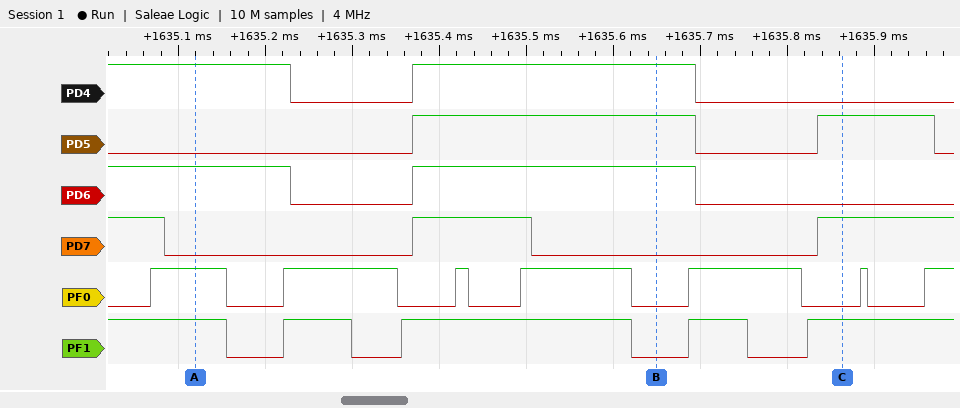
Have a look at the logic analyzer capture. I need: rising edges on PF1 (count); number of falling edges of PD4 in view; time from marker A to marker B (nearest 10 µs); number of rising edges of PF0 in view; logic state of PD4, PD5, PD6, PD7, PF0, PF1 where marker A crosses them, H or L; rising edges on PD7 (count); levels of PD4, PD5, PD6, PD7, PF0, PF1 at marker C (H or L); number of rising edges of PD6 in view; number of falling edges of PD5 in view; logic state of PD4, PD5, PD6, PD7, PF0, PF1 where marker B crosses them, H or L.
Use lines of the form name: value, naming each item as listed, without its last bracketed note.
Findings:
rising edges on PF1: 4
number of falling edges of PD4 in view: 2
time from marker A to marker B: 530 µs
number of rising edges of PF0 in view: 7
logic state of PD4, PD5, PD6, PD7, PF0, PF1 where marker A crosses them, H or L: PD4=H, PD5=L, PD6=H, PD7=L, PF0=H, PF1=H
rising edges on PD7: 2
levels of PD4, PD5, PD6, PD7, PF0, PF1 at marker C: PD4=L, PD5=H, PD6=L, PD7=H, PF0=L, PF1=H
number of rising edges of PD6 in view: 1
number of falling edges of PD5 in view: 2
logic state of PD4, PD5, PD6, PD7, PF0, PF1 where marker B crosses them, H or L: PD4=H, PD5=H, PD6=H, PD7=L, PF0=L, PF1=L
